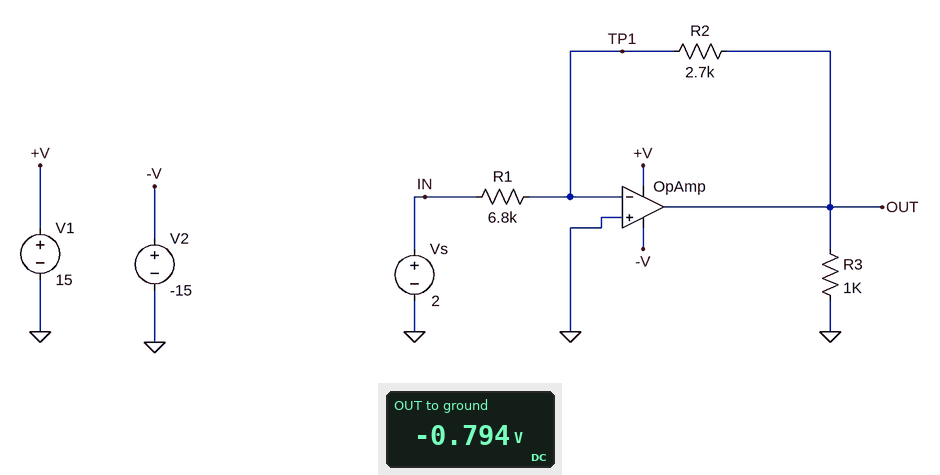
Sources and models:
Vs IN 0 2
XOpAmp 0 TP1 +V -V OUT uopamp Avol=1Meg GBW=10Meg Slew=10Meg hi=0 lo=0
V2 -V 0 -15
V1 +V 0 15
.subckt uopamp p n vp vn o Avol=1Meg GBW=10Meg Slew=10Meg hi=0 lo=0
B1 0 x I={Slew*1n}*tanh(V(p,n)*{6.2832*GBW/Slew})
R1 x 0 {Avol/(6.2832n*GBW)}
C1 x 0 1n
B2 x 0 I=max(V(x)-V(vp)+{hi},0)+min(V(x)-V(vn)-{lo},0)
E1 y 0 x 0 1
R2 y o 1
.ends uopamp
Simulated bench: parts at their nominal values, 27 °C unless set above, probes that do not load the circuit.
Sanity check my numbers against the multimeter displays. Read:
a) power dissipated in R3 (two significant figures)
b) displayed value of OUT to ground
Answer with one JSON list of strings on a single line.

["630 µW", "-0.794 V"]
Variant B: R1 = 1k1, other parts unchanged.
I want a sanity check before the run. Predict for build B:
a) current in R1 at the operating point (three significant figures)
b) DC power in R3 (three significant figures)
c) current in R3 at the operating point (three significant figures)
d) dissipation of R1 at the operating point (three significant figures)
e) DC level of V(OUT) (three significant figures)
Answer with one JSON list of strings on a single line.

["1.82 mA", "24.1 mW", "4.91 mA", "3.64 mW", "-4.91 V"]
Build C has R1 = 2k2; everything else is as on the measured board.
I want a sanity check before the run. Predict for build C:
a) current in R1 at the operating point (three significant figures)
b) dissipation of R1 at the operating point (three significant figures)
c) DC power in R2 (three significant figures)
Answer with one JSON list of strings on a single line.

["909 µA", "1.82 mW", "2.23 mW"]
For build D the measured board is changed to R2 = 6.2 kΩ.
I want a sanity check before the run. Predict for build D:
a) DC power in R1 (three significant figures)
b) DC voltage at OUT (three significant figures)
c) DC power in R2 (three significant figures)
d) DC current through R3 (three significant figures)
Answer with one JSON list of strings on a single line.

["588 µW", "-1.82 V", "536 µW", "1.82 mA"]
